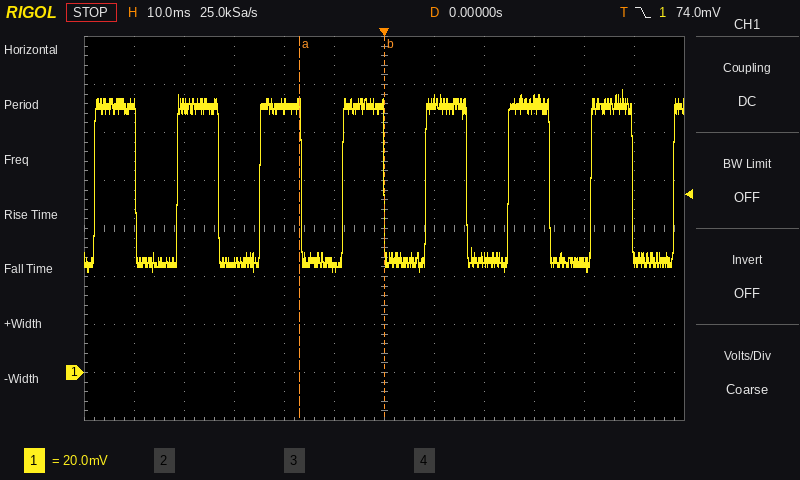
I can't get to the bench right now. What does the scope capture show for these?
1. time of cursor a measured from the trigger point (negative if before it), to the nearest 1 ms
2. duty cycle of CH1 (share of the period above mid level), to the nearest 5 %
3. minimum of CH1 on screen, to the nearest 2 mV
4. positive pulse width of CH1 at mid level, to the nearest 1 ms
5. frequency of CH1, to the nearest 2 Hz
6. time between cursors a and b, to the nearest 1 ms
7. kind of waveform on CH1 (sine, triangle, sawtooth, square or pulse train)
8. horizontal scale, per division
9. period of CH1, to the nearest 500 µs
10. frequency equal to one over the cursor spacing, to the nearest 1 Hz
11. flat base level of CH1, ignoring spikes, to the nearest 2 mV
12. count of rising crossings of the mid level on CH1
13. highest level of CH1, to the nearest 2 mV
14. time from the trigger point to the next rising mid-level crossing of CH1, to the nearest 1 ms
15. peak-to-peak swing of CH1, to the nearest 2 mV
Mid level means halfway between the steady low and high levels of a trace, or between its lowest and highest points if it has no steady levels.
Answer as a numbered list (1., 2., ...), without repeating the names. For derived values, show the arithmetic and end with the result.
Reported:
1. -17 ms
2. 8 ms / 16.5 ms ≈ 48.5 %, so 50 % to the nearest 5 %
3. 42 mV
4. 8 ms
5. 1 / 16.5 ms ≈ 60.6 Hz, so 60 Hz to the nearest 2 Hz
6. 17 ms
7. square
8. 10 ms
9. 16.5 ms
10. 1 / 17 ms ≈ 59 Hz
11. 46 mV
12. 8
13. 118 mV
14. 8 ms
15. 118 mV − (42 mV) = 76 mV
